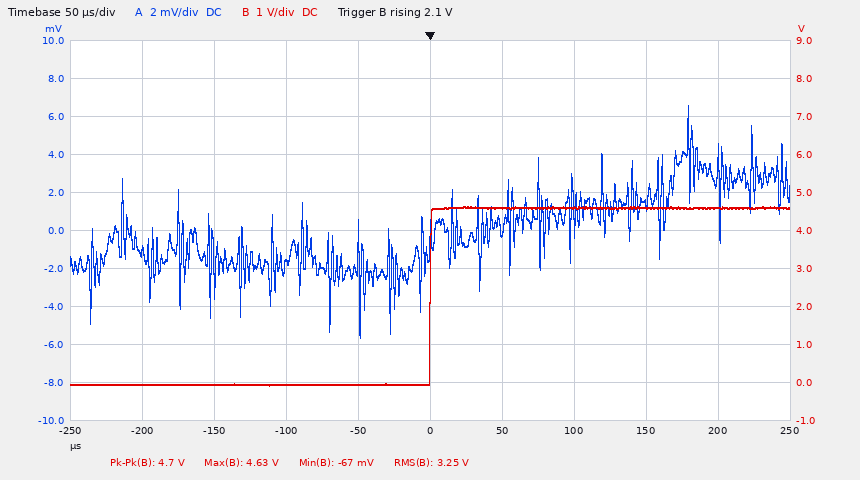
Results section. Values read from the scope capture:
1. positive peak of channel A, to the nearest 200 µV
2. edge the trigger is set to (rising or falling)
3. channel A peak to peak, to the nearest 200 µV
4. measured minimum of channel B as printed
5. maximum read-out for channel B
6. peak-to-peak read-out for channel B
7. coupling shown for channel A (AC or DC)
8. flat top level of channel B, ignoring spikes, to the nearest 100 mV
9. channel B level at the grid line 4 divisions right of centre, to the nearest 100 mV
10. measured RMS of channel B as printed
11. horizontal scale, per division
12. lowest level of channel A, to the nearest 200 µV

6.6 mV
rising
12.2 mV
-67 mV
4.63 V
4.7 V
DC
4.6 V
4.6 V
3.25 V
50 µs
-5.6 mV
